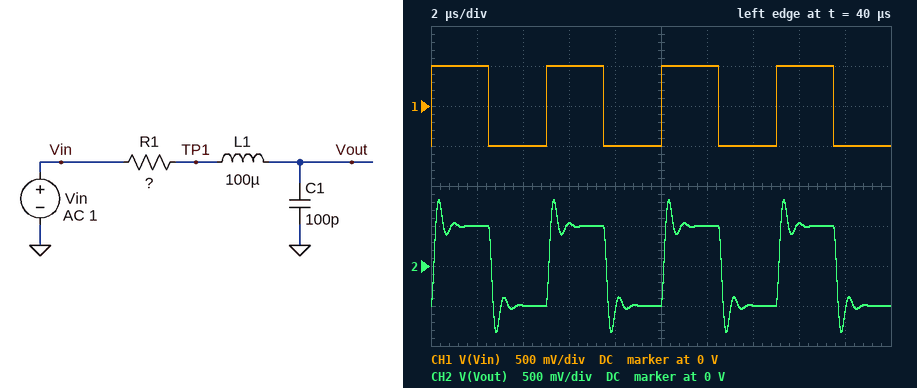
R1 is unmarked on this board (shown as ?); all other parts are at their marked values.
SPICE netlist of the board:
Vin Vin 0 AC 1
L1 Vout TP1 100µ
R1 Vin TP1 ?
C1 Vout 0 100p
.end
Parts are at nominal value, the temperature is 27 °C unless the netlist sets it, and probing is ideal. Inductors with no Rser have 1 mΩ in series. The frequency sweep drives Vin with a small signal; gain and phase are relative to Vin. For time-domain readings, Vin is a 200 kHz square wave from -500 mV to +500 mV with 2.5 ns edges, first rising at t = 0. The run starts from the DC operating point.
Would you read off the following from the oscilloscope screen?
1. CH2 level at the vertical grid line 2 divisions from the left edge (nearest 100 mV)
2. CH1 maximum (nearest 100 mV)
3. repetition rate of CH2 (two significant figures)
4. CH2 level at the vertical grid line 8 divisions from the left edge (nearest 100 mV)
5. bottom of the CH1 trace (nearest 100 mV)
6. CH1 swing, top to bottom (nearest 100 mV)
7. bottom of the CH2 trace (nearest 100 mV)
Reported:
-500 mV
500 mV
200 kHz
500 mV
-500 mV
1.0 V
-800 mV
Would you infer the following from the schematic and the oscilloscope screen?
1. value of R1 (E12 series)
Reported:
680 Ω
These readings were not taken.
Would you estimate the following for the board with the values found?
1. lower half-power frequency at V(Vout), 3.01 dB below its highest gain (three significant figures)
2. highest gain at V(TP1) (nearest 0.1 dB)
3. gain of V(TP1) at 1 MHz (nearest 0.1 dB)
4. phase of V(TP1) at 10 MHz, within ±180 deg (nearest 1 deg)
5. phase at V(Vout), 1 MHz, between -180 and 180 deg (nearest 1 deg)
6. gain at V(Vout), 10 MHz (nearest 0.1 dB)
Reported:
572 kHz
0 dB
-1.8 dB
6 deg
-35 deg
-31.8 dB
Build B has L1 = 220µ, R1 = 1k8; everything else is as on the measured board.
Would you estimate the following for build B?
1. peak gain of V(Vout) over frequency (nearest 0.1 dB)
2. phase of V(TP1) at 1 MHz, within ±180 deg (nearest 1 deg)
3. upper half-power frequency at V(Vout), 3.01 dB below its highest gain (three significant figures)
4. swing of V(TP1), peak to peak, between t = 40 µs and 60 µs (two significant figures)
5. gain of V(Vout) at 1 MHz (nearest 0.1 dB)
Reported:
0.3 dB
-83 deg
1.19 MHz
1.1 V
-1.1 dB
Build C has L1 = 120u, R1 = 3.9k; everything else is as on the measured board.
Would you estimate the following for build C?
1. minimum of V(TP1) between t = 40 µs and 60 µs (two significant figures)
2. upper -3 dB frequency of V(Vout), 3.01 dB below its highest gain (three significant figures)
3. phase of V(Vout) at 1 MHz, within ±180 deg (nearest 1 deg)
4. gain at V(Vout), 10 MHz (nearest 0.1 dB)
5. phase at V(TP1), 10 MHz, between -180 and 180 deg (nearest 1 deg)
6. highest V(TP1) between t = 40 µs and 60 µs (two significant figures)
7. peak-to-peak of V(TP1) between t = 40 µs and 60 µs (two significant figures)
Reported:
-500 mV
443 kHz
-78 deg
-34.4 dB
28 deg
500 mV
1.0 V
